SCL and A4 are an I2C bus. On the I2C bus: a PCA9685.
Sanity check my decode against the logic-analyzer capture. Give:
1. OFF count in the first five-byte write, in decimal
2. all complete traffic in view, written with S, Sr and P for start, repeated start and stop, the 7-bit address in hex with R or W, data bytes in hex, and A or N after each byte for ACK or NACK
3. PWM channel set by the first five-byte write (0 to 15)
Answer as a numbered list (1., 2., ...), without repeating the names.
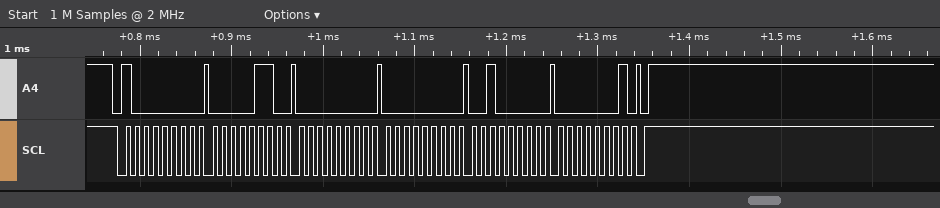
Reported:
1. 288
2. S 40W A 06 A 00 A 00 A 20 A 01 A P
3. 0
